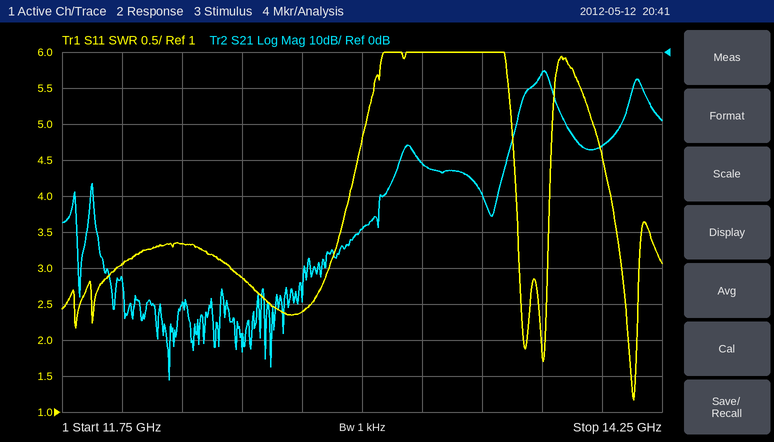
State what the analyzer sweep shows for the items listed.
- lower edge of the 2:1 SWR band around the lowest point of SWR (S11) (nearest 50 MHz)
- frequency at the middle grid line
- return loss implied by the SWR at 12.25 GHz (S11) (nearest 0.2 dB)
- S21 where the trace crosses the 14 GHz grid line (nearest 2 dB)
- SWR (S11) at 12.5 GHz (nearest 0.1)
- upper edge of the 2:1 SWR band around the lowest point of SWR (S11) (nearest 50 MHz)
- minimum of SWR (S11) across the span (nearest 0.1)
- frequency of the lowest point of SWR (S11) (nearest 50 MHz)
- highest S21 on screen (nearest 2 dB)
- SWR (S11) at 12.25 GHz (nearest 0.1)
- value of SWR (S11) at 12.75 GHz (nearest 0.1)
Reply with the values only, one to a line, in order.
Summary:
14.10 GHz
13 GHz
5.4 dB
-26 dB
2.9
14.15 GHz
1.2
14.15 GHz
-6 dB
3.3
2.4
